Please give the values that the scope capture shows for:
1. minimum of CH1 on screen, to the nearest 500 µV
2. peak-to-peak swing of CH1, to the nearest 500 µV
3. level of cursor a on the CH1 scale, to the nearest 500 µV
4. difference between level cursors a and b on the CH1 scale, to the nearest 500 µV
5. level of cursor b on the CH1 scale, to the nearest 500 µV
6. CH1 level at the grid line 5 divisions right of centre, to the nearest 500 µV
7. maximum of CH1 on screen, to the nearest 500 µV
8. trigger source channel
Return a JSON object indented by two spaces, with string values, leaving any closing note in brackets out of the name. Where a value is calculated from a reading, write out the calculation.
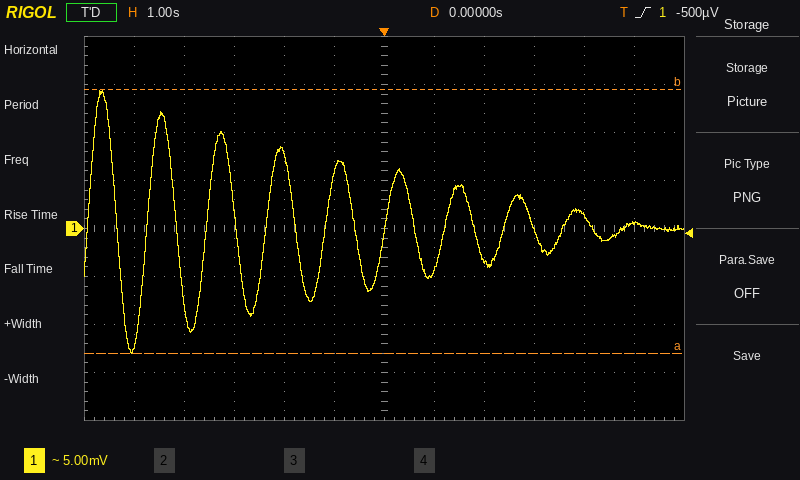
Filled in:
{
  "minimum of CH1 on screen, to the nearest 500 µV": "-13.0 mV",
  "peak-to-peak swing of CH1, to the nearest 500 µV": "14.5 mV − (-13.0 mV) = 27.5 mV",
  "level of cursor a on the CH1 scale, to the nearest 500 µV": "-13.0 mV",
  "difference between level cursors a and b on the CH1 scale, to the nearest 500 µV": "27.5 mV",
  "level of cursor b on the CH1 scale, to the nearest 500 µV": "14.5 mV",
  "CH1 level at the grid line 5 divisions right of centre, to the nearest 500 µV": "500 µV",
  "maximum of CH1 on screen, to the nearest 500 µV": "14.5 mV",
  "trigger source channel": "CH1"
}
